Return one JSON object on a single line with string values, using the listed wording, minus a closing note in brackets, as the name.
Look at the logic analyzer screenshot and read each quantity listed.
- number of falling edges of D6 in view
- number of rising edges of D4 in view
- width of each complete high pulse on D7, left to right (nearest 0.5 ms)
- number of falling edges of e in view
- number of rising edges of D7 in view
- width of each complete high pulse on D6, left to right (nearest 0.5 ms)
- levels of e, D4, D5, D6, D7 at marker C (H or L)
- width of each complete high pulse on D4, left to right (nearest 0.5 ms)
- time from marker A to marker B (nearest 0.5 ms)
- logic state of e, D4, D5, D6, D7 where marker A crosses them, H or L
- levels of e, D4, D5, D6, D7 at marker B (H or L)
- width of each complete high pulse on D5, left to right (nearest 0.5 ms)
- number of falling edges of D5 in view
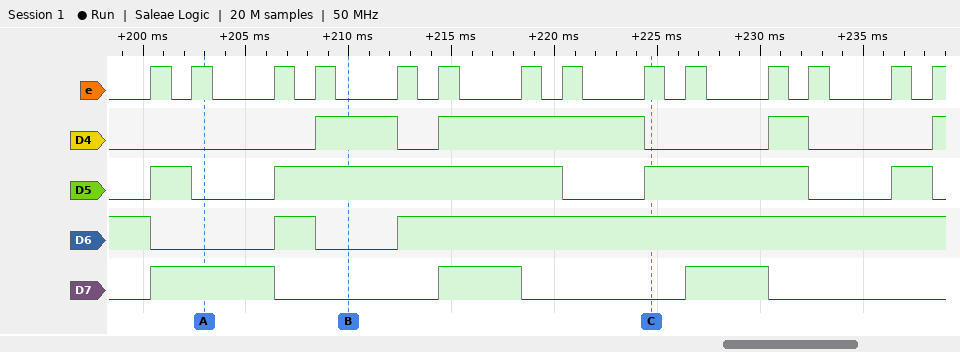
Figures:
{"number of falling edges of D6 in view": "2", "number of rising edges of D4 in view": "4", "width of each complete high pulse on D7, left to right": "6 ms, 4 ms, 4 ms", "number of falling edges of e in view": "13", "number of rising edges of D7 in view": "3", "width of each complete high pulse on D6, left to right": "2 ms", "levels of e, D4, D5, D6, D7 at marker C": "e=H, D4=L, D5=H, D6=H, D7=L", "width of each complete high pulse on D4, left to right": "4 ms, 10 ms, 2 ms", "time from marker A to marker B": "7 ms", "logic state of e, D4, D5, D6, D7 where marker A crosses them, H or L": "e=H, D4=L, D5=L, D6=L, D7=H", "levels of e, D4, D5, D6, D7 at marker B": "e=L, D4=H, D5=H, D6=L, D7=L", "width of each complete high pulse on D5, left to right": "2 ms, 14 ms, 8 ms, 2 ms", "number of falling edges of D5 in view": "4"}
